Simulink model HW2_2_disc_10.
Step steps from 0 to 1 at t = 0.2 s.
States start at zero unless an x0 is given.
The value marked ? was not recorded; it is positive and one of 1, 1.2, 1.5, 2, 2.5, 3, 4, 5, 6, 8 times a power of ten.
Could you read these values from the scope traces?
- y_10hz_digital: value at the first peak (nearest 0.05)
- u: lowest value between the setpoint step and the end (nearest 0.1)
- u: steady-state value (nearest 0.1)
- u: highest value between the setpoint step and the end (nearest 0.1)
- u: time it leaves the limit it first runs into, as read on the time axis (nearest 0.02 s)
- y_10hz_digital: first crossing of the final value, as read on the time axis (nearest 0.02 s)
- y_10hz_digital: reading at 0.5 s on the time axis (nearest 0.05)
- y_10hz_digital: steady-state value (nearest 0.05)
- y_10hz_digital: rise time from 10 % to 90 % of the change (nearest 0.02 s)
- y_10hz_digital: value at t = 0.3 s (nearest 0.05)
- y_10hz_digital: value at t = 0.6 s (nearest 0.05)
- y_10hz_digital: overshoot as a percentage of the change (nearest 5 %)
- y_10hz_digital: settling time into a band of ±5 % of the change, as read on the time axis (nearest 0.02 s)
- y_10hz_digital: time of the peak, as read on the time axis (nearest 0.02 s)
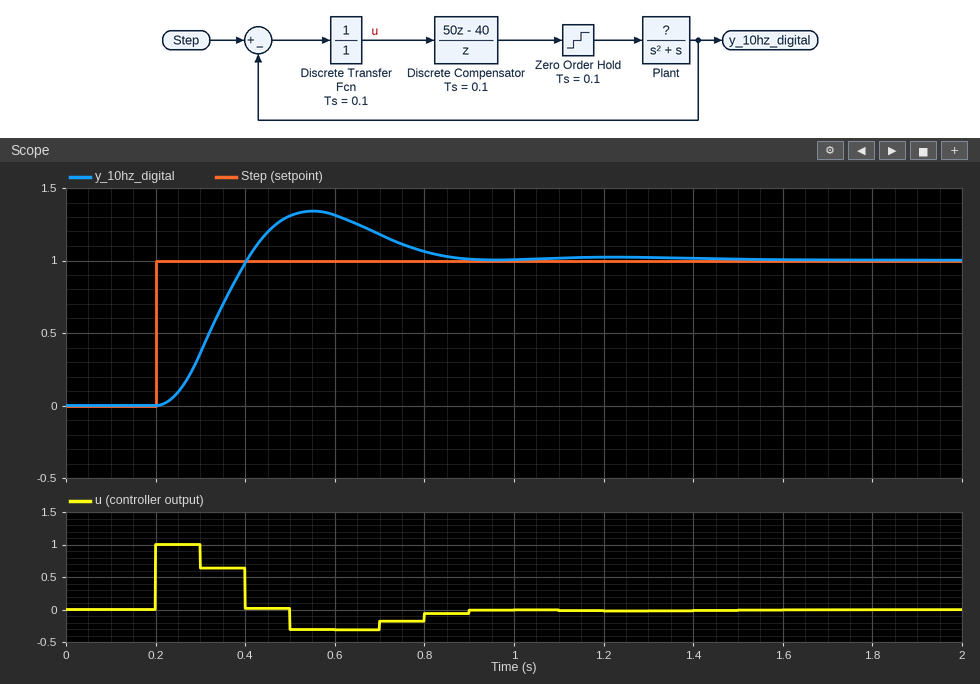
1.35
-0.3
0.0
1.0
0.30 s
0.40 s
1.30
1.00
0.14 s
0.35
1.30
35 %
0.82 s
0.56 s
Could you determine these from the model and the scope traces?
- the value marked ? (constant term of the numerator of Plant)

1.5
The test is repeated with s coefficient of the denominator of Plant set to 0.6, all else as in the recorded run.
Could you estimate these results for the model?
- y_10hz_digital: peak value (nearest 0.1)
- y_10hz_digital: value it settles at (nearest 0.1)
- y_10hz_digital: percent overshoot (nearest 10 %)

1.4
1.0
40 %
